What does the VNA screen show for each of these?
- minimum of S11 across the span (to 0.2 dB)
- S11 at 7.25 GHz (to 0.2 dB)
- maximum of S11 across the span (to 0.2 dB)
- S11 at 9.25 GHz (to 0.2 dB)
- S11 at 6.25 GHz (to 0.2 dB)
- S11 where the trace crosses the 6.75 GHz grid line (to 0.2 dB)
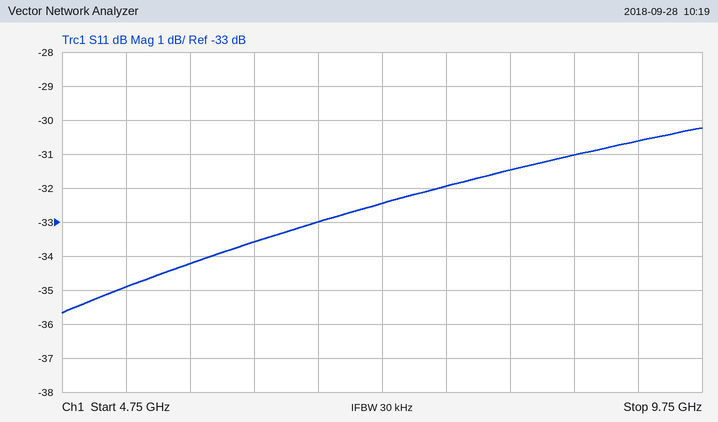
-35.6 dB
-32.4 dB
-30.2 dB
-30.6 dB
-33.6 dB
-33.0 dB
